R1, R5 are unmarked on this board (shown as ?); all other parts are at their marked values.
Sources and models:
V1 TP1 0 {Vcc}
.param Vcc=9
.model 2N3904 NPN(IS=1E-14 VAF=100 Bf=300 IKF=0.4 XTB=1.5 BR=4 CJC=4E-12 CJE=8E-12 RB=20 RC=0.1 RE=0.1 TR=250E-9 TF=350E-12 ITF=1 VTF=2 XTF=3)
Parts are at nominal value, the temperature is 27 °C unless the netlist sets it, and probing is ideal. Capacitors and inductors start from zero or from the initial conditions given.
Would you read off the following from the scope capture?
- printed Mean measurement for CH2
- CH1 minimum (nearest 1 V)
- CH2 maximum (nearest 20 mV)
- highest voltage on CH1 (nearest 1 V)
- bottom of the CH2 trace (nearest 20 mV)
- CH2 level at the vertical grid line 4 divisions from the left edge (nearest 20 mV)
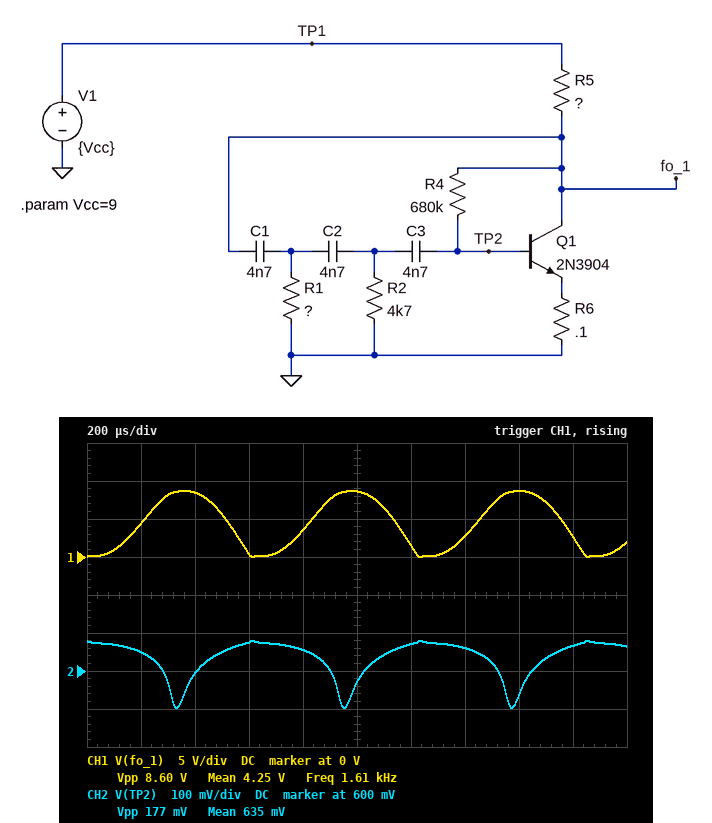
635 mV
0 V
680 mV
9 V
500 mV
660 mV
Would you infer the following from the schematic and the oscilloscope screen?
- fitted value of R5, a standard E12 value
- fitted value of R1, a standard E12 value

4.7 kΩ
12 kΩ
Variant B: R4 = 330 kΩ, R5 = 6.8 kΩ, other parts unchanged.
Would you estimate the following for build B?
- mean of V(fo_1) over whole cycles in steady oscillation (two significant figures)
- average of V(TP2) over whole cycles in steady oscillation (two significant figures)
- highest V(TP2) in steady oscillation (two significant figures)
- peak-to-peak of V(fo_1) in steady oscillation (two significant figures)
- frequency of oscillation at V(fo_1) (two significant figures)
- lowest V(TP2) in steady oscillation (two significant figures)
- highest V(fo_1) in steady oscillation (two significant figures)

2.3 V
650 mV
670 mV
4.5 V
1.9 kHz
640 mV
4.6 V
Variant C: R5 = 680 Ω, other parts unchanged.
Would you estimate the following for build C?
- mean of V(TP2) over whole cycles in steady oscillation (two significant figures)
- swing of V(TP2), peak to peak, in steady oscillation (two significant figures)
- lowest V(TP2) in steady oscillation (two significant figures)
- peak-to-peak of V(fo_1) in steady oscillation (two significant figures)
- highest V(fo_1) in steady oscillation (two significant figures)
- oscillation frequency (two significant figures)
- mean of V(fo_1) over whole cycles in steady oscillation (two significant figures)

680 mV
35 mV
660 mV
2.2 V
8.1 V
2.1 kHz
7.0 V
